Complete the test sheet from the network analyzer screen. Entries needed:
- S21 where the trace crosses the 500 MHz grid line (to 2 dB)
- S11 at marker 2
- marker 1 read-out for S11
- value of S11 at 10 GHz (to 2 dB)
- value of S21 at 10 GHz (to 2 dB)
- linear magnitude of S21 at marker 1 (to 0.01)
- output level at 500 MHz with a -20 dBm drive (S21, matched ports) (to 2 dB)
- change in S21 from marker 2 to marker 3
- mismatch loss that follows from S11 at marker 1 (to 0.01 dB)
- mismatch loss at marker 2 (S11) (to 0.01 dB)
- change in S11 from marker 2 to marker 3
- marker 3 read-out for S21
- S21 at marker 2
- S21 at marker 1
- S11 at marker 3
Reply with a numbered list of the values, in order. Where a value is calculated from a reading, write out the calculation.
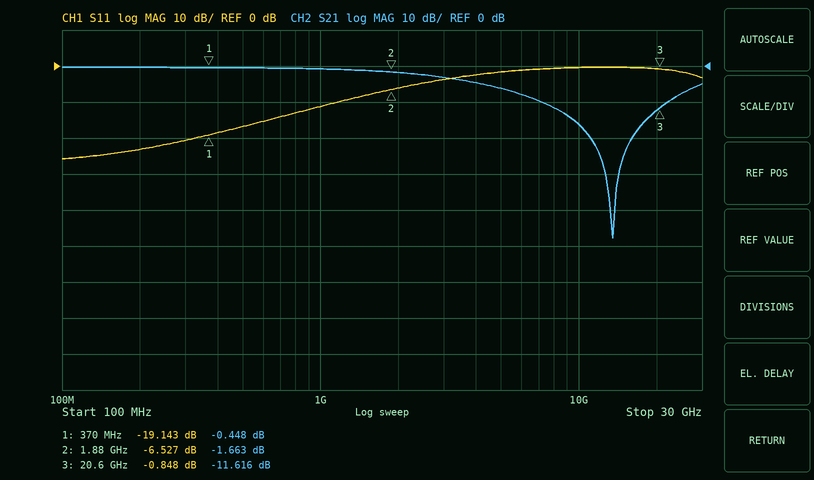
1. 0 dB
2. -6.527 dB
3. -19.143 dB
4. 0 dB
5. -16 dB
6. 10^(-0.448/20) ≈ 0.95
7. -20 dBm + (0 dB) = -20 dBm
8. -11.616 − (-1.663) = -9.953 dB
9. −10 log10(1 − 10^(-19.143/10)) ≈ 0.05 dB
10. −10 log10(1 − 10^(-6.527/10)) ≈ 1.09 dB
11. -0.848 − (-6.527) = 5.679 dB
12. -11.616 dB
13. -1.663 dB
14. -0.448 dB
15. -0.848 dB
